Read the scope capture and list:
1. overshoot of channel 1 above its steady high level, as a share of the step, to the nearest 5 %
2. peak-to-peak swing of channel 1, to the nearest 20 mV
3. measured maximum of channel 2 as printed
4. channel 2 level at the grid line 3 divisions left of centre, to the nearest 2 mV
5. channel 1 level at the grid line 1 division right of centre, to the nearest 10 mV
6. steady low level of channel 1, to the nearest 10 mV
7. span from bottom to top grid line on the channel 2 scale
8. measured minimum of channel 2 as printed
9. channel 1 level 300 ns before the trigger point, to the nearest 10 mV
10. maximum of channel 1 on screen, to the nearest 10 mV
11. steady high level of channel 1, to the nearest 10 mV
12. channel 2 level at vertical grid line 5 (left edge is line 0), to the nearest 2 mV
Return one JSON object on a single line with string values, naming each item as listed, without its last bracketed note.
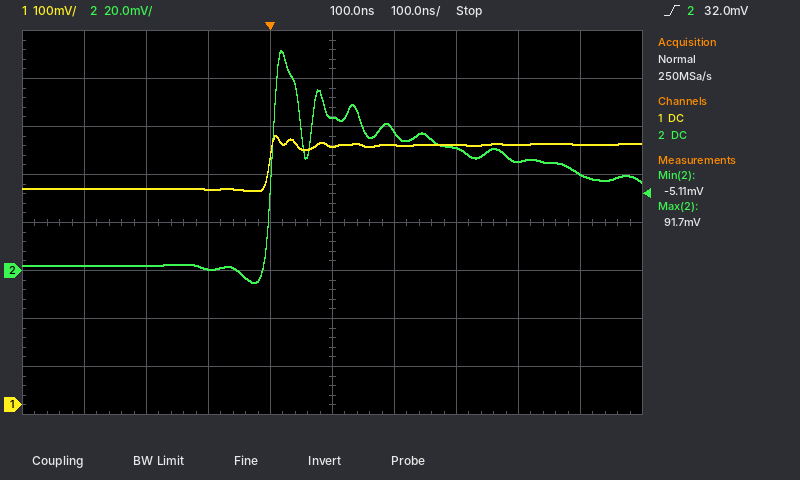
{"overshoot of channel 1 above its steady high level, as a share of the step, to the nearest 5 %": "20 %", "peak-to-peak swing of channel 1, to the nearest 20 mV": "120 mV", "measured maximum of channel 2 as printed": "91.7 mV", "channel 2 level at the grid line 3 divisions left of centre, to the nearest 2 mV": "2 mV", "channel 1 level at the grid line 1 division right of centre, to the nearest 10 mV": "540 mV", "steady low level of channel 1, to the nearest 10 mV": "450 mV", "span from bottom to top grid line on the channel 2 scale": "160 mV", "measured minimum of channel 2 as printed": "-5.11 mV", "channel 1 level 300 ns before the trigger point, to the nearest 10 mV": "450 mV", "maximum of channel 1 on screen, to the nearest 10 mV": "560 mV", "steady high level of channel 1, to the nearest 10 mV": "540 mV", "channel 2 level at vertical grid line 5 (left edge is line 0), to the nearest 2 mV": "64 mV"}
